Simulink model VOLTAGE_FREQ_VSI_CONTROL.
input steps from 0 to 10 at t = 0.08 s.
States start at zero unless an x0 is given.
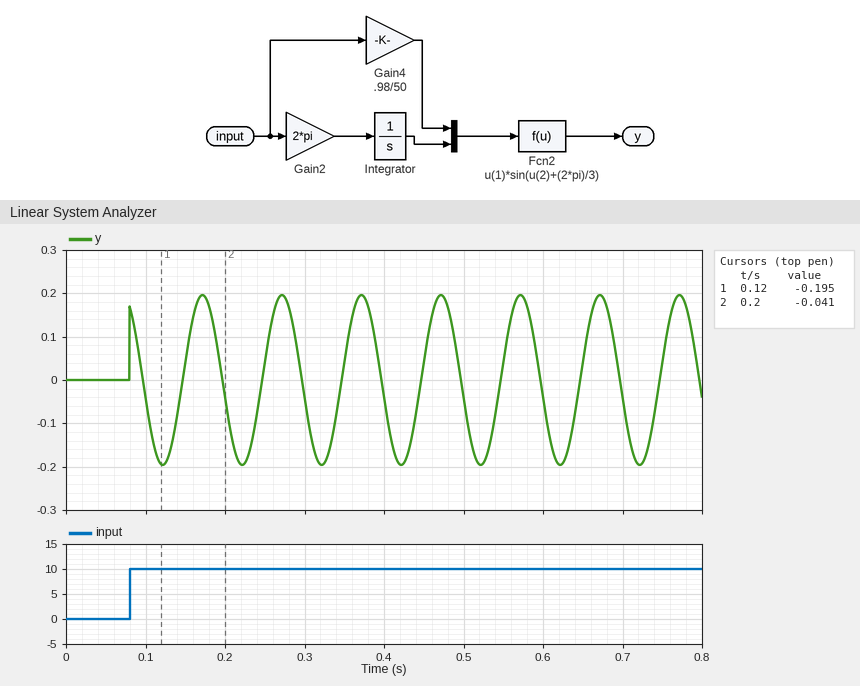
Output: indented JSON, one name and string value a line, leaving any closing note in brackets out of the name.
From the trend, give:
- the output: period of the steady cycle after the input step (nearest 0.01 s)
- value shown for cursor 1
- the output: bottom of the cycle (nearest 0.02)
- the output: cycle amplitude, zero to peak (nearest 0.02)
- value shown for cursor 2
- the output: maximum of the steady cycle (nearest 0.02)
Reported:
{
  "the output: period of the steady cycle after the input step": "0.10 s",
  "value shown for cursor 1": "-0.195",
  "the output: bottom of the cycle": "-0.20",
  "the output: cycle amplitude, zero to peak": "0.20",
  "value shown for cursor 2": "-0.041",
  "the output: maximum of the steady cycle": "0.20"
}
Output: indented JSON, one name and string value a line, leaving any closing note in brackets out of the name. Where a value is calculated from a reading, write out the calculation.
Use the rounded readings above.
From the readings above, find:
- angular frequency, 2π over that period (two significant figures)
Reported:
{
  "angular frequency, 2π over that period": "2π / 0.1 = 63 rad/s"
}
